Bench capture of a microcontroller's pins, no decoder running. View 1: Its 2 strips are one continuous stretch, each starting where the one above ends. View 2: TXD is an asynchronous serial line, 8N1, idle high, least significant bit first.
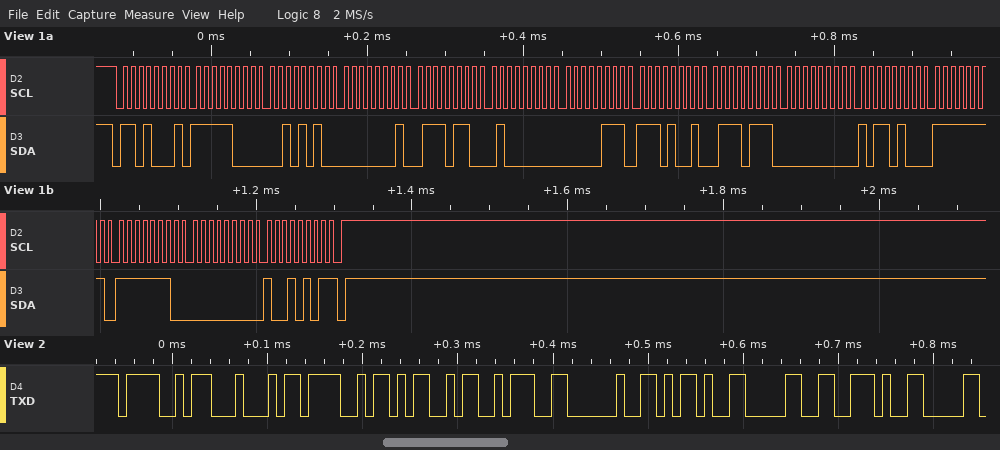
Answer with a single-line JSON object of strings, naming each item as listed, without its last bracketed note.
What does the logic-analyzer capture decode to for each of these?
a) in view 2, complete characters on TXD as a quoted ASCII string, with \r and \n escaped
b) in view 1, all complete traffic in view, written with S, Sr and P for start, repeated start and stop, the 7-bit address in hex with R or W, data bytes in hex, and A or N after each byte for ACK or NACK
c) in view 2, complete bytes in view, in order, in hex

{"in view 2, complete characters on TXD as a quoted ASCII string, with \\r and \\n escaped": "\"ODOM: -0.\"", "in view 1, all complete traffic in view, written with S, Sr and P for start, repeated start and stop, the 7-bit address in hex with R or W, data bytes in hex, and A or N after each byte for ACK or NACK": "S 68R A F8 A 2A A 01 A 76 A 40 A 07 A E9 A 77 A 00 A B4 A FF A FE A 00 A 95 N P", "in view 2, complete bytes in view, in order, in hex": "4F 44 4F 4D 3A 20 2D 30 2E"}
